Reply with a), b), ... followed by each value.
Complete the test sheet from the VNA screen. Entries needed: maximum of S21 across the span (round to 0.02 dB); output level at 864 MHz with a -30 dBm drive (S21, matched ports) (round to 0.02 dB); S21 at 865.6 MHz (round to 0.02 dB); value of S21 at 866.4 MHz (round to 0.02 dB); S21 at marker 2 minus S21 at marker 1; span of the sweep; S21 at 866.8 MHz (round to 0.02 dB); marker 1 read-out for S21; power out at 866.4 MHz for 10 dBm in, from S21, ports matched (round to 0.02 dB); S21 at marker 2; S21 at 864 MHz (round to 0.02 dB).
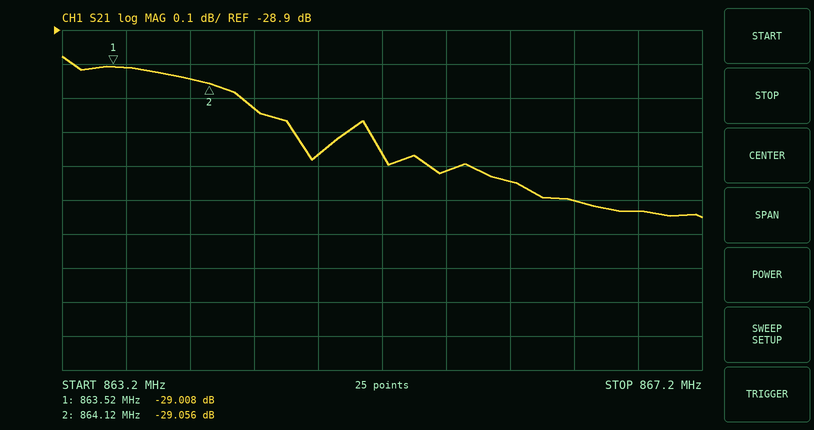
a) -28.98 dB
b) -59.04 dBm
c) -29.32 dB
d) -29.40 dB
e) -0.048 dB
f) 4 MHz
g) -29.44 dB
h) -29.008 dB
i) -19.40 dBm
j) -29.056 dB
k) -29.04 dB
